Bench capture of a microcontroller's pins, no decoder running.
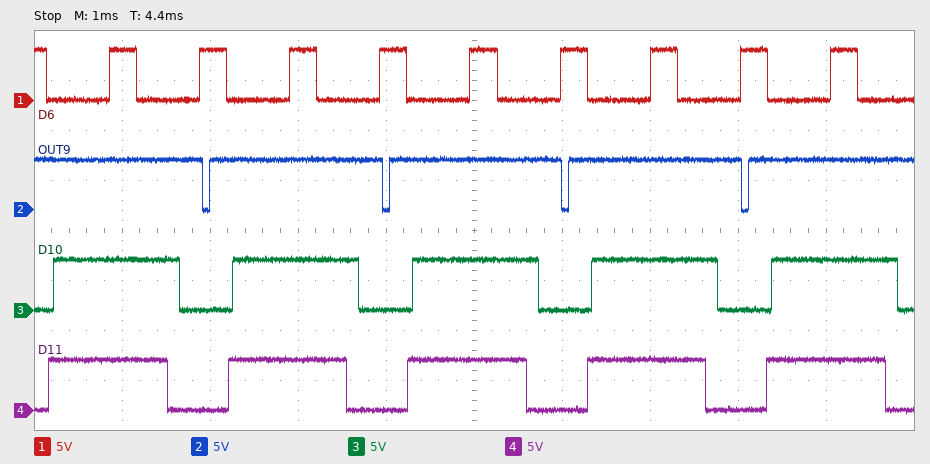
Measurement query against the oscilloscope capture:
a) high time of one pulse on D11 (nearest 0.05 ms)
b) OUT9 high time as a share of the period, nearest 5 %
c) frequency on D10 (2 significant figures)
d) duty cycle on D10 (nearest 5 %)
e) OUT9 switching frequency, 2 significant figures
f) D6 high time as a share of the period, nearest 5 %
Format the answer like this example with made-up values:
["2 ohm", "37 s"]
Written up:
["1.35 ms", "95 %", "490 Hz", "70 %", "490 Hz", "30 %"]
